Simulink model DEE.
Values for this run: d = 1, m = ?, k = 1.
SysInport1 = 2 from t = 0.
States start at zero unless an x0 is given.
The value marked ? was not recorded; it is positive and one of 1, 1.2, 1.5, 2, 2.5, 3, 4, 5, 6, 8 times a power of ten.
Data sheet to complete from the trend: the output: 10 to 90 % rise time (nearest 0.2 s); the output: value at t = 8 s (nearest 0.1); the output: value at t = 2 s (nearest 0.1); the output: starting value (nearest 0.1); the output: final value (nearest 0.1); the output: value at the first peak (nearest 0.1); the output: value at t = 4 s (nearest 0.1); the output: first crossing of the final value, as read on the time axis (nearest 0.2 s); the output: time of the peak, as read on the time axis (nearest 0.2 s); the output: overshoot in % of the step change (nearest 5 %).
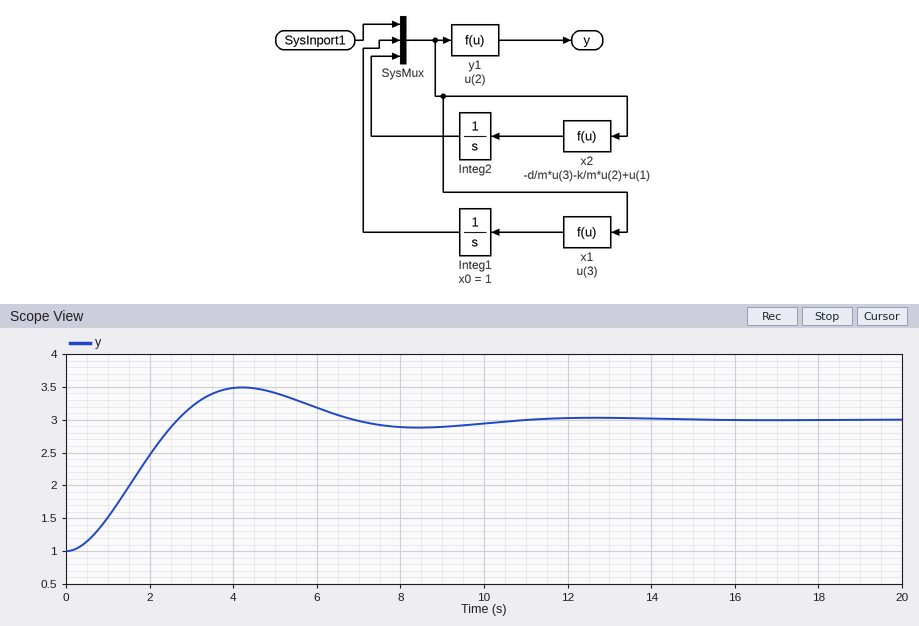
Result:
1.8 s
2.9
2.5
1.0
3.0
3.5
3.5
2.6 s
4.2 s
25 %
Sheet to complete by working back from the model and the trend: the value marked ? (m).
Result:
1.5
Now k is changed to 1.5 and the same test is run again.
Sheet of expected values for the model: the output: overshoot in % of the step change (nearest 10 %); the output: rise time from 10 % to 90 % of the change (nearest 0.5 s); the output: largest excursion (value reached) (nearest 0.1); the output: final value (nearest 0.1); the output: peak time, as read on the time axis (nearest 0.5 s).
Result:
30 %
1.5 s
2.3
2.0
3.5 s
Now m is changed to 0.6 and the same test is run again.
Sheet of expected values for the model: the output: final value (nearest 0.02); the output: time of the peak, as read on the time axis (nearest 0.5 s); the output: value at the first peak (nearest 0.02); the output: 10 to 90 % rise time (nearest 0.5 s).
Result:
1.20
3.0 s
1.22
1.5 s
